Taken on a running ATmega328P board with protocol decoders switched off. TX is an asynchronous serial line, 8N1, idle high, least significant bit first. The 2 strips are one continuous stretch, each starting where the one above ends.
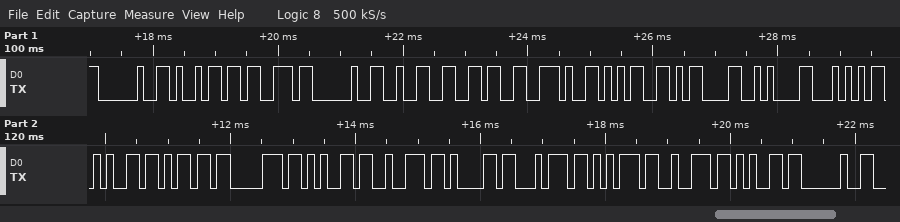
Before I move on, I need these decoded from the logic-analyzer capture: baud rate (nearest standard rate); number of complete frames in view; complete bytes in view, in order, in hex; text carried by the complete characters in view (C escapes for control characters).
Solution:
9600 baud
22
20 69 73 20 32 36 2E 35 0D 0A 54 65 6D 70 65 72 61 74 75 72 65 20
" is 26.5\r\nTemperature "
